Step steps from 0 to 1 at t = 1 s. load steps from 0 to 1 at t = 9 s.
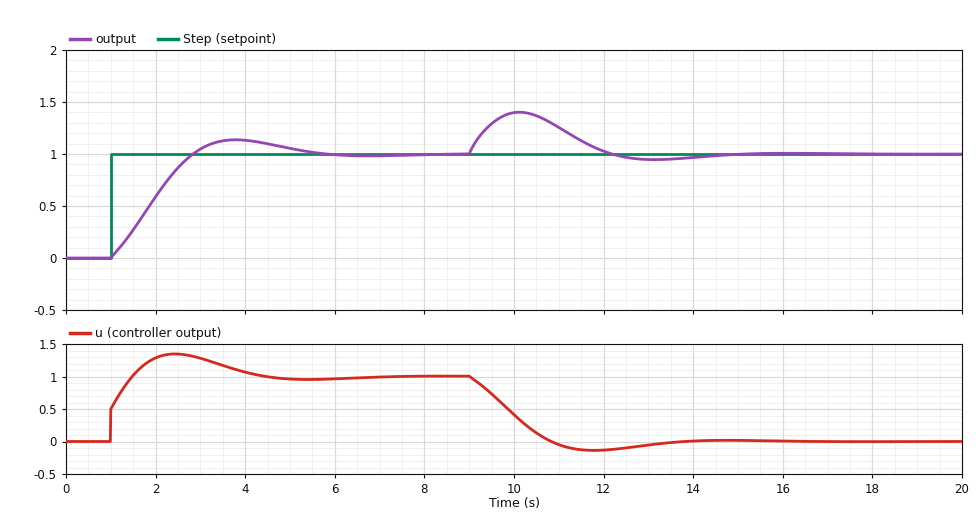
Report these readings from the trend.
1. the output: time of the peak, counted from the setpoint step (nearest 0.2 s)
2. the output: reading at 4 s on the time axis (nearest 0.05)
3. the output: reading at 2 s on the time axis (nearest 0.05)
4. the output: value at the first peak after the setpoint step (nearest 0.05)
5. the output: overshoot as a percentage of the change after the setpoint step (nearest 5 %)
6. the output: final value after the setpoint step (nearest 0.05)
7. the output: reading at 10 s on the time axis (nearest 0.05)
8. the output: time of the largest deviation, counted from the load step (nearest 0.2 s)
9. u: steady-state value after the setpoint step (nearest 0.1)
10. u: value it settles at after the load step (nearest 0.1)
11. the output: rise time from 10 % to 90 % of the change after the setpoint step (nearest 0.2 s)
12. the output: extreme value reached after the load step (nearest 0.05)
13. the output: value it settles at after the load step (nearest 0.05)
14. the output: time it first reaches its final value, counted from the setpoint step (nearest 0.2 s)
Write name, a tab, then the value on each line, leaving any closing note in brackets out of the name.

the output: time of the peak, counted from the setpoint step	2.8 s
the output: reading at 4 s on the time axis	1.15
the output: reading at 2 s on the time axis	0.60
the output: value at the first peak after the setpoint step	1.15
the output: overshoot as a percentage of the change after the setpoint step	15 %
the output: final value after the setpoint step	1.00
the output: reading at 10 s on the time axis	1.40
the output: time of the largest deviation, counted from the load step	1.2 s
u: steady-state value after the setpoint step	1.0
u: value it settles at after the load step	0.0
the output: rise time from 10 % to 90 % of the change after the setpoint step	1.4 s
the output: extreme value reached after the load step	1.40
the output: value it settles at after the load step	1.00
the output: time it first reaches its final value, counted from the setpoint step	1.8 s
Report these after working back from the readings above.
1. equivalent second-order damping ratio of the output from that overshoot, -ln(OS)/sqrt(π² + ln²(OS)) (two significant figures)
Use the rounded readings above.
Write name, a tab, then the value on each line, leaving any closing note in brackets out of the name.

equivalent second-order damping ratio of the output from that overshoot, -ln(OS)/sqrt(π² + ln²(OS))	0.52
